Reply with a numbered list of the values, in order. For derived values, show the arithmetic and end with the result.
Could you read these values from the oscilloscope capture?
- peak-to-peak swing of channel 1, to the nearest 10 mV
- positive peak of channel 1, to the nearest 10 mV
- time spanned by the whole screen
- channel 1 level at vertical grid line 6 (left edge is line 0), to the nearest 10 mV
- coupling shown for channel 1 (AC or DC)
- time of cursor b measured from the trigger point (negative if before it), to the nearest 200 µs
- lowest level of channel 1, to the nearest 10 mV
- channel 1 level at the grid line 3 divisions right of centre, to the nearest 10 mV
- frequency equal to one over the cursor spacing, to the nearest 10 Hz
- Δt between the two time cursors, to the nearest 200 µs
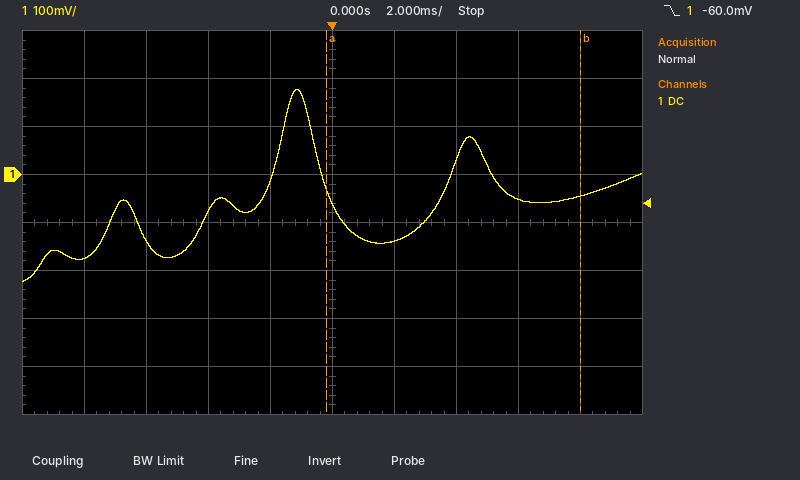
1. 180 mV − (-220 mV) = 400 mV
2. 180 mV
3. 20 ms
4. -140 mV
5. DC
6. +8.0 ms
7. -220 mV
8. -50 mV
9. 1 / 8.2 ms ≈ 120 Hz
10. 8.2 ms
